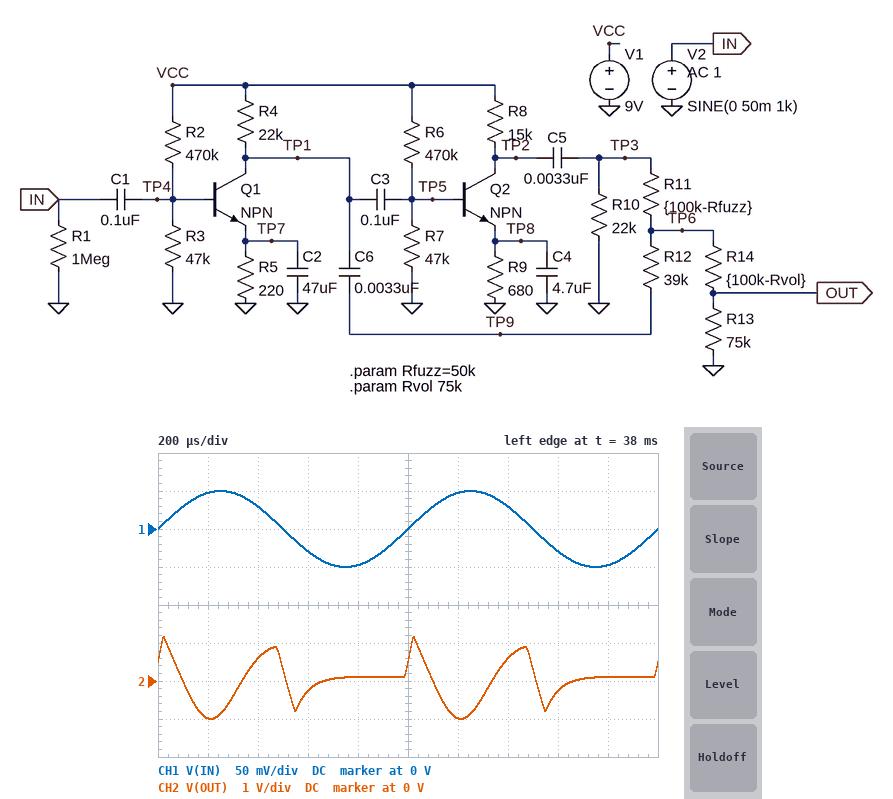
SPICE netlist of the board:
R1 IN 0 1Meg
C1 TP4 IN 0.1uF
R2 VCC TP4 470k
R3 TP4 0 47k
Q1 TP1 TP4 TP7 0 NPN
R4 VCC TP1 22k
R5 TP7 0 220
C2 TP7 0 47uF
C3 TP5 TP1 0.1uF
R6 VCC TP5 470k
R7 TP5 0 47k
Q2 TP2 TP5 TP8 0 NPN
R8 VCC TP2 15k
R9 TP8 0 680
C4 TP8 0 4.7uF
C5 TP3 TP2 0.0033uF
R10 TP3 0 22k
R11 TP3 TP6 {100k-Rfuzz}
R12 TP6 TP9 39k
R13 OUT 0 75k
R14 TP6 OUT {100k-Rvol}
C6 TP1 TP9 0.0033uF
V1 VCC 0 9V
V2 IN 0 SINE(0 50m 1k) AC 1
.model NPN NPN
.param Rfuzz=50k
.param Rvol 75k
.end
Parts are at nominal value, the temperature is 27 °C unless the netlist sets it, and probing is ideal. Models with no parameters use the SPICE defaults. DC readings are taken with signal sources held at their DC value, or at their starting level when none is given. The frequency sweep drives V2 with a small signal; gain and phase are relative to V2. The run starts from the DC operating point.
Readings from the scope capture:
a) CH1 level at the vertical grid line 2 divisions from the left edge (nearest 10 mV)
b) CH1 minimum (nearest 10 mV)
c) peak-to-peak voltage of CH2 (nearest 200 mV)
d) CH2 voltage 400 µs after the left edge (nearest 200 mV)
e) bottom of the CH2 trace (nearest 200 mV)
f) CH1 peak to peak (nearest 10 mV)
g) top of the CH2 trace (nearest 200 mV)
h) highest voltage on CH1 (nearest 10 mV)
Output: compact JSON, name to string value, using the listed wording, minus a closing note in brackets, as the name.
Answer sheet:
{"CH1 level at the vertical grid line 2 divisions from the left edge": "30 mV", "CH1 minimum": "-50 mV", "peak-to-peak voltage of CH2": "2.2 V", "CH2 voltage 400 µs after the left edge": "600 mV", "bottom of the CH2 trace": "-1.0 V", "CH1 peak to peak": "100 mV", "top of the CH2 trace": "1.2 V", "highest voltage on CH1": "50 mV"}
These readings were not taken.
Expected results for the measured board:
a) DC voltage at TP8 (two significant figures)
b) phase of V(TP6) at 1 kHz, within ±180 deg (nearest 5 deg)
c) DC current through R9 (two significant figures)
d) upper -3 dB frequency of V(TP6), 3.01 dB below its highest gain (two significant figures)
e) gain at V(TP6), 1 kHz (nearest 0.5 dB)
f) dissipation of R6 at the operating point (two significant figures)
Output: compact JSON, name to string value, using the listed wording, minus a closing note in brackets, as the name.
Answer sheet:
{"DC voltage at TP8": "65 mV", "phase of V(TP6) at 1 kHz, within ±180 deg": "0 deg", "DC current through R9": "95 µA", "upper -3 dB frequency of V(TP6), 3.01 dB below its highest gain": "1.1 kHz", "gain at V(TP6), 1 kHz": "47.5 dB", "dissipation of R6 at the operating point": "140 µW"}
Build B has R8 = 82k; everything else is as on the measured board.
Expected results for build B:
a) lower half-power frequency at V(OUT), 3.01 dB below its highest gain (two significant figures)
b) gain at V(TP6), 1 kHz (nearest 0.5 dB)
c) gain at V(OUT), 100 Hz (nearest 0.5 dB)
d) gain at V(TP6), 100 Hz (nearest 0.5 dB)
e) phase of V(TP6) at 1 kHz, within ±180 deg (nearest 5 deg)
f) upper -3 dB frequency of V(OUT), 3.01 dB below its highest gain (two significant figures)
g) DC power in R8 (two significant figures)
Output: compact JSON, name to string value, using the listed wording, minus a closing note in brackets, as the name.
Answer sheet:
{"lower half-power frequency at V(OUT), 3.01 dB below its highest gain": "210 Hz", "gain at V(TP6), 1 kHz": "49.0 dB", "gain at V(OUT), 100 Hz": "41.0 dB", "gain at V(TP6), 100 Hz": "43.5 dB", "phase of V(TP6) at 1 kHz, within ±180 deg": "-30 deg", "upper -3 dB frequency of V(OUT), 3.01 dB below its highest gain": "350 Hz", "DC power in R8": "730 µW"}
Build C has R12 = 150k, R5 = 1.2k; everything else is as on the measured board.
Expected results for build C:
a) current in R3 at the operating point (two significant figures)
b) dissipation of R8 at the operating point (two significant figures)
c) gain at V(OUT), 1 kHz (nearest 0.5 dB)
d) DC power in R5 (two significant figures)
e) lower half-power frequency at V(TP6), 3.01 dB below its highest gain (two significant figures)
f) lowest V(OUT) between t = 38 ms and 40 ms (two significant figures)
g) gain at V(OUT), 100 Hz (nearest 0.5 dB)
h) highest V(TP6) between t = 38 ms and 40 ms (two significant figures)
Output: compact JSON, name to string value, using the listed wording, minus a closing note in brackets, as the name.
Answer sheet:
{"current in R3 at the operating point": "17 µA", "dissipation of R8 at the operating point": "130 µW", "gain at V(OUT), 1 kHz": "42.5 dB", "DC power in R5": "5.8 µW", "lower half-power frequency at V(TP6), 3.01 dB below its highest gain": "510 Hz", "lowest V(OUT) between t = 38 ms and 40 ms": "-1.8 V", "gain at V(OUT), 100 Hz": "21.5 dB", "highest V(TP6) between t = 38 ms and 40 ms": "2.1 V"}
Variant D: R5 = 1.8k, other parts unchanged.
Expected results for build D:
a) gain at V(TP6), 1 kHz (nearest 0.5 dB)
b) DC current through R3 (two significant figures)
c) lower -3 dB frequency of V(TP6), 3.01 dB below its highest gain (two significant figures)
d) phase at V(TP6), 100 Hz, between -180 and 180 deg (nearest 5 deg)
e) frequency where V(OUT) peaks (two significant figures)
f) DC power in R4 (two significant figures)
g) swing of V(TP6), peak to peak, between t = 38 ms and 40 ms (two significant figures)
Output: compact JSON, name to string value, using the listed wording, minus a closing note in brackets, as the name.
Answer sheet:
{"gain at V(TP6), 1 kHz": "39.0 dB", "DC current through R3": "17 µA", "lower -3 dB frequency of V(TP6), 3.01 dB below its highest gain": "340 Hz", "phase at V(TP6), 100 Hz, between -180 and 180 deg": "170 deg", "frequency where V(OUT) peaks": "550 Hz", "DC power in R4": "63 µW", "swing of V(TP6), peak to peak, between t = 38 ms and 40 ms": "2.3 V"}
